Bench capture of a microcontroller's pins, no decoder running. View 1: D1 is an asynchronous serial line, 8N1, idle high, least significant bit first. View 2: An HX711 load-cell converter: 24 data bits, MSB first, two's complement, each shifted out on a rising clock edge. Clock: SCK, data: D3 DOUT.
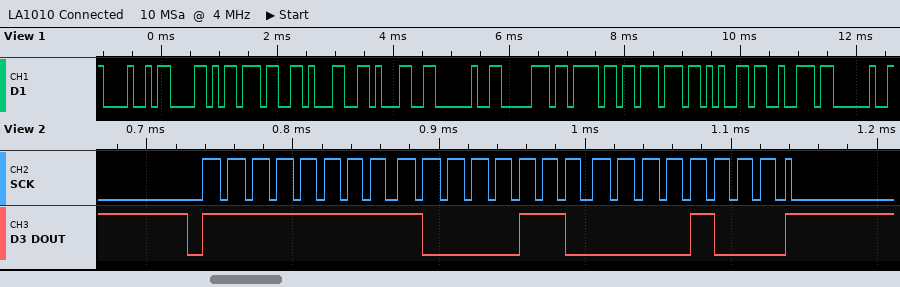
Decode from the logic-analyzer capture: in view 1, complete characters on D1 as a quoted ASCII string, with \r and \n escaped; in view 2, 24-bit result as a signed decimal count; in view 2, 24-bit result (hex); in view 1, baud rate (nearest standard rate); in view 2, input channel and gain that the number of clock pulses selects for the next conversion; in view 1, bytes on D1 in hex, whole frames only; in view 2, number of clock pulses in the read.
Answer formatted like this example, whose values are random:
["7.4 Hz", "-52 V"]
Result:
["\"HX711 power \"", "-31224", "0xFF8608", "9600 baud", "channel A, gain 128", "48 58 37 31 31 20 70 6F 77 65 72 20", "25"]
